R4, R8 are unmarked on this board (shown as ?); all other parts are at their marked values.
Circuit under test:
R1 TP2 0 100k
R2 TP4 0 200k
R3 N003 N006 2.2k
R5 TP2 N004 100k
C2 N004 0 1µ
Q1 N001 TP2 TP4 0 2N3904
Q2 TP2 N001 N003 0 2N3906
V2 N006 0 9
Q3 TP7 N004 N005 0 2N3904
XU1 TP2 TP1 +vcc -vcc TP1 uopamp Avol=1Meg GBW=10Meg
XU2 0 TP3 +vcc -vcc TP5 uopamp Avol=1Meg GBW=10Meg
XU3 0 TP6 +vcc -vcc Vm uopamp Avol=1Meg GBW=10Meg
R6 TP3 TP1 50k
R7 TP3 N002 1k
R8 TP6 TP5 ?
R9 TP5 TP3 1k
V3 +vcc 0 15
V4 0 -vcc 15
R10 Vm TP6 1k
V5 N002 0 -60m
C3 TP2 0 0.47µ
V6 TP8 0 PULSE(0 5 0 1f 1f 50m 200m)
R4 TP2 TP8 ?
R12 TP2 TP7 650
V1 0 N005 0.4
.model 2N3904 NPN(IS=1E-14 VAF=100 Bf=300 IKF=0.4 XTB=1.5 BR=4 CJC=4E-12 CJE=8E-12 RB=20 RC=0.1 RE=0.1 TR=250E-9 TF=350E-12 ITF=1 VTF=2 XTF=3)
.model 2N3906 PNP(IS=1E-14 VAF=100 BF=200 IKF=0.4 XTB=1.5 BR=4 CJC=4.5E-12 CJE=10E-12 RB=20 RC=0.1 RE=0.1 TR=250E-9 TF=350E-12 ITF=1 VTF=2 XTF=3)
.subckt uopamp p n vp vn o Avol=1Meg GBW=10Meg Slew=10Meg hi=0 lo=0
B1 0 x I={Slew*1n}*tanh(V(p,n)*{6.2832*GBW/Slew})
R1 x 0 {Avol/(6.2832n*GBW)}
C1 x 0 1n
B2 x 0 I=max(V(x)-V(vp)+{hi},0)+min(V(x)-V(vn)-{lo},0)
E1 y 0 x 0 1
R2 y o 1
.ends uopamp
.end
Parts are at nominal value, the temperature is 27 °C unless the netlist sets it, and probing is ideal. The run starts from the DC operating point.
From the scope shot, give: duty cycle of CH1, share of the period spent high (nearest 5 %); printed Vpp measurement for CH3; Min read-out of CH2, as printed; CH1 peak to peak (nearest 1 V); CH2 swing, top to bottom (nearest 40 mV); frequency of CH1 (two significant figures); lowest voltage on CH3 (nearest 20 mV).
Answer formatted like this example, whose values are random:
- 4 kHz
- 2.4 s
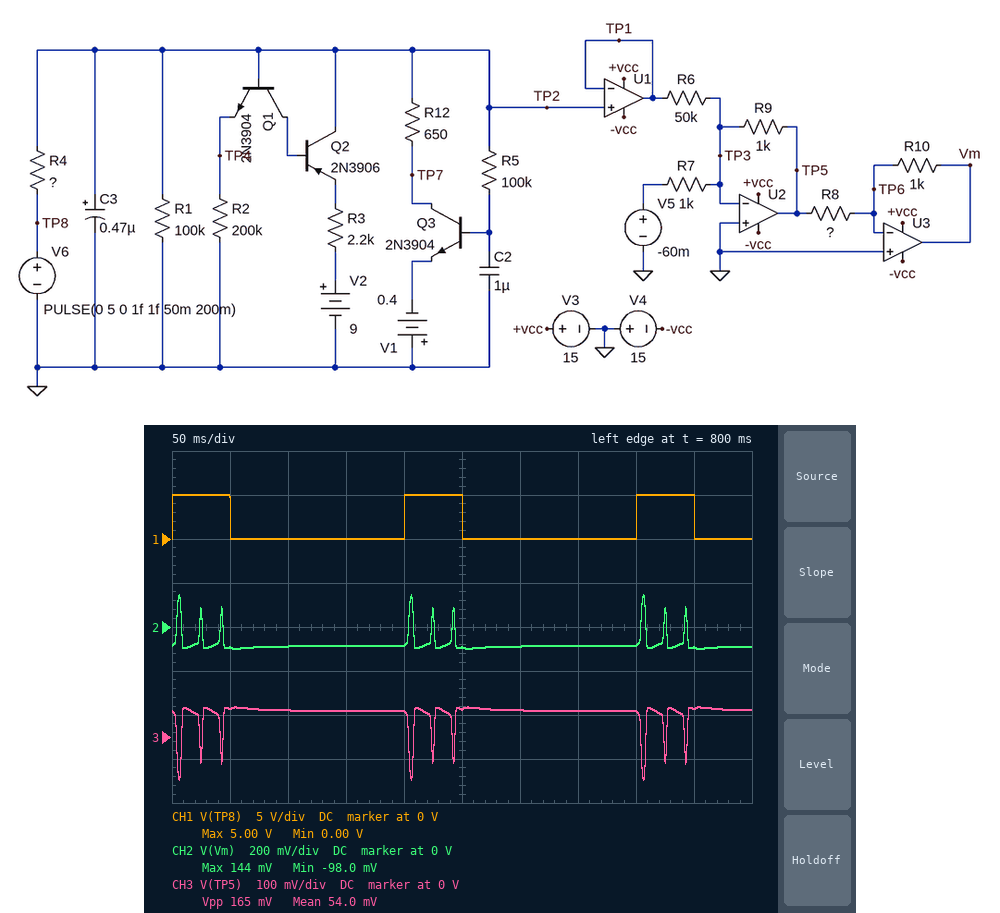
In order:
- 25 %
- 165 mV
- -98.0 mV
- 5 V
- 240 mV
- 5.0 Hz
- -100 mV
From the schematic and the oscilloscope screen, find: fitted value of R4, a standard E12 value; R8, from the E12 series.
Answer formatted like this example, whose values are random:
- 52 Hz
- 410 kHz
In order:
- 56 kΩ
- 680 Ω
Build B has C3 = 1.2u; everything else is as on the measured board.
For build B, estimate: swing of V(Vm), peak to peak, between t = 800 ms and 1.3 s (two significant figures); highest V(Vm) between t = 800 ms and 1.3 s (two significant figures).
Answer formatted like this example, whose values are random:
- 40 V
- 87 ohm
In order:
- 210 mV
- 110 mV
